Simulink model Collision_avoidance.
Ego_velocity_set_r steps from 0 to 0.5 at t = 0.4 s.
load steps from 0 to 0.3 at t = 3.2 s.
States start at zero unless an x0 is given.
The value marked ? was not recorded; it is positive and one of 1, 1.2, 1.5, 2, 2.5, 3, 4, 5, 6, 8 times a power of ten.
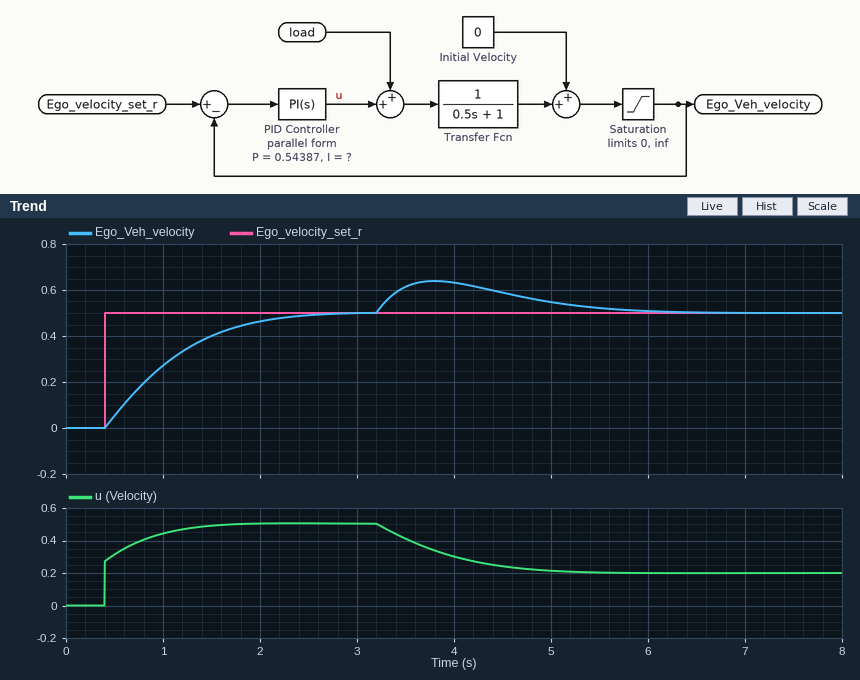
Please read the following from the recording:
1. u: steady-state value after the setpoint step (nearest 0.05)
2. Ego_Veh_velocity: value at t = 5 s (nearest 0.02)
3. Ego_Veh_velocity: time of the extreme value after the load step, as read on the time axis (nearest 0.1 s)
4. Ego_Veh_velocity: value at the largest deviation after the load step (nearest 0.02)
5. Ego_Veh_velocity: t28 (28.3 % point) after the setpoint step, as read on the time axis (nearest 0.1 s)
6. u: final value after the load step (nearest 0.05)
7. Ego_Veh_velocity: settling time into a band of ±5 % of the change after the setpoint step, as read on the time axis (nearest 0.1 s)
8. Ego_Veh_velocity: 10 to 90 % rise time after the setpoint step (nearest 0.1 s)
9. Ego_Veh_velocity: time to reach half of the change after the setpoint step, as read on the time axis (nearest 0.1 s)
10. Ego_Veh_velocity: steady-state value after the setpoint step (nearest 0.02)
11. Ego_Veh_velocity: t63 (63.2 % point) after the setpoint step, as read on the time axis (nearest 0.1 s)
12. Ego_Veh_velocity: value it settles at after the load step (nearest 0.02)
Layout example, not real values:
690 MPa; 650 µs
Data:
0.50; 0.54; 3.8 s; 0.64; 0.7 s; 0.20; 2.2 s; 1.4 s; 0.9 s; 0.50; 1.1 s; 0.50
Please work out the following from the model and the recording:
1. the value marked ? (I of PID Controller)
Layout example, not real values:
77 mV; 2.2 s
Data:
1.5
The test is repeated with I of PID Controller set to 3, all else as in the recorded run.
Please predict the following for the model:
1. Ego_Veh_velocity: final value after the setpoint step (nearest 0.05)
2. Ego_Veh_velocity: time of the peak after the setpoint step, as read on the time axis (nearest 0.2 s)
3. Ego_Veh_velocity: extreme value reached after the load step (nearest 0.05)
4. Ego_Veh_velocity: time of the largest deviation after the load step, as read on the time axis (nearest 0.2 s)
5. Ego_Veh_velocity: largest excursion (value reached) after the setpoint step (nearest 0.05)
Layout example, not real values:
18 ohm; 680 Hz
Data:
0.50; 1.8 s; 0.60; 3.6 s; 0.55
